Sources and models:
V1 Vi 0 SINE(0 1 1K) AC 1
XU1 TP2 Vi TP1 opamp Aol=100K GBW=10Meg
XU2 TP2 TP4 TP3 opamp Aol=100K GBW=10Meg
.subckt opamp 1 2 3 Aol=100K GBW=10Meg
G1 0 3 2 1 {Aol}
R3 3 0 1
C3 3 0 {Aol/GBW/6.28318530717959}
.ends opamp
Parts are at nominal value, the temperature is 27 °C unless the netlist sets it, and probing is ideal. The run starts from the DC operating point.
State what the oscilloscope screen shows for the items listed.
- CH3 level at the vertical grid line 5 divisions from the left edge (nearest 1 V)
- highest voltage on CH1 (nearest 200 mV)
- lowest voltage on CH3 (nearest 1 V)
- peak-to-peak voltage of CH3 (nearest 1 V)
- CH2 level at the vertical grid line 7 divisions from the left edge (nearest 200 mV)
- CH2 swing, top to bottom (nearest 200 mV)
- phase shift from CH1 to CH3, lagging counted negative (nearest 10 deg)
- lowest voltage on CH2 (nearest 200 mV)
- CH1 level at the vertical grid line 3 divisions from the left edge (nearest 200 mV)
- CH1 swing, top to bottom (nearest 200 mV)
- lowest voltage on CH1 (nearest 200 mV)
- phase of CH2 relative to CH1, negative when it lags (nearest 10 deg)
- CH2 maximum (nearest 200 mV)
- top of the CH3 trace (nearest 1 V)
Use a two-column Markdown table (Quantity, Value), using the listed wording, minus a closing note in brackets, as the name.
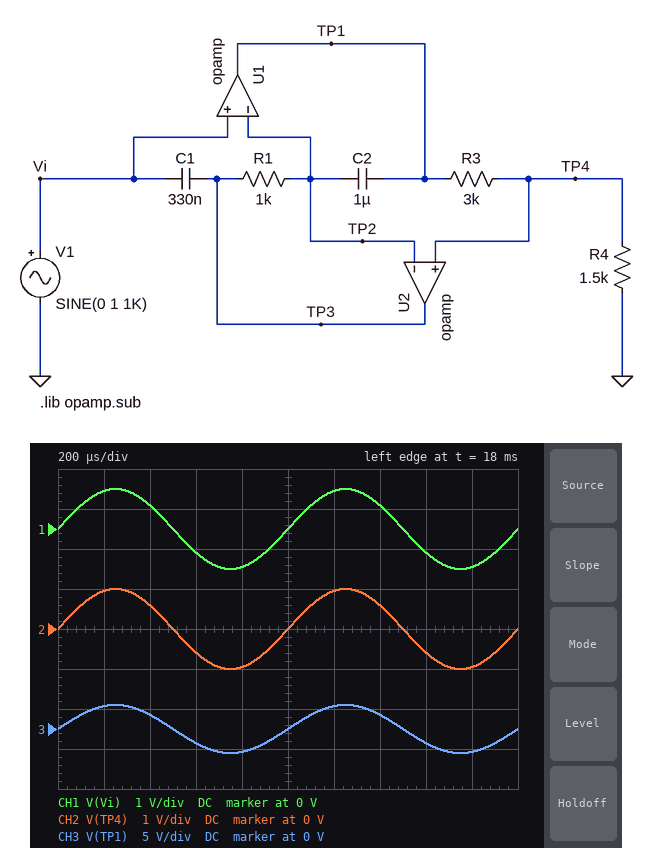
| Quantity | Value |
|---|---|
| CH3 level at the vertical grid line 5 divisions from the left edge | 0 V |
| highest voltage on CH1 | 1.0 V |
| lowest voltage on CH3 | -3 V |
| peak-to-peak voltage of CH3 | 6 V |
| CH2 level at the vertical grid line 7 divisions from the left edge | 600 mV |
| CH2 swing, top to bottom | 2.0 V |
| phase shift from CH1 to CH3, lagging counted negative | 0 deg |
| lowest voltage on CH2 | -1.0 V |
| CH1 level at the vertical grid line 3 divisions from the left edge | -600 mV |
| CH1 swing, top to bottom | 2.0 V |
| lowest voltage on CH1 | -1.0 V |
| phase of CH2 relative to CH1, negative when it lags | 0 deg |
| CH2 maximum | 1.0 V |
| top of the CH3 trace | 3 V |
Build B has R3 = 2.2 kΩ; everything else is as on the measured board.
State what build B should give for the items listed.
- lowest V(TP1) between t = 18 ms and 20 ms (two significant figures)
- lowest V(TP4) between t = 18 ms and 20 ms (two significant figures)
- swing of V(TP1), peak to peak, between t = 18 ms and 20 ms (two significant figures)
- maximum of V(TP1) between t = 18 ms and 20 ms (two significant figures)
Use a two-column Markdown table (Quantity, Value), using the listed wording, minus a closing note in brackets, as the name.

| Quantity | Value |
|---|---|
| lowest V(TP1) between t = 18 ms and 20 ms | -2.5 V |
| lowest V(TP4) between t = 18 ms and 20 ms | -1.0 V |
| swing of V(TP1), peak to peak, between t = 18 ms and 20 ms | 4.9 V |
| maximum of V(TP1) between t = 18 ms and 20 ms | 2.5 V |
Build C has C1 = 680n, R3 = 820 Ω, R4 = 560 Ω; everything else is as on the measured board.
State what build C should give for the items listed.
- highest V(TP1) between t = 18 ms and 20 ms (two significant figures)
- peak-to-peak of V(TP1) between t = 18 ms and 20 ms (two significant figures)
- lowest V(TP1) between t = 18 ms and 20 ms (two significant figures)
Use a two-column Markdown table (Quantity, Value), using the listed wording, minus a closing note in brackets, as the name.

| Quantity | Value |
|---|---|
| highest V(TP1) between t = 18 ms and 20 ms | 2.5 V |
| peak-to-peak of V(TP1) between t = 18 ms and 20 ms | 4.9 V |
| lowest V(TP1) between t = 18 ms and 20 ms | -2.5 V |
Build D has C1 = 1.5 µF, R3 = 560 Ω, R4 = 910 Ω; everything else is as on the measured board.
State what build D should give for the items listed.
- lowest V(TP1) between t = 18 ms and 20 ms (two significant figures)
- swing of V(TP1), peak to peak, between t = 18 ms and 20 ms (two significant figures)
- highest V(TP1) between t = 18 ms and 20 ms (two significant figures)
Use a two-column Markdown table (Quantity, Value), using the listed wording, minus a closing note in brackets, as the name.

| Quantity | Value |
|---|---|
| lowest V(TP1) between t = 18 ms and 20 ms | -1.6 V |
| swing of V(TP1), peak to peak, between t = 18 ms and 20 ms | 3.2 V |
| highest V(TP1) between t = 18 ms and 20 ms | 1.6 V |
